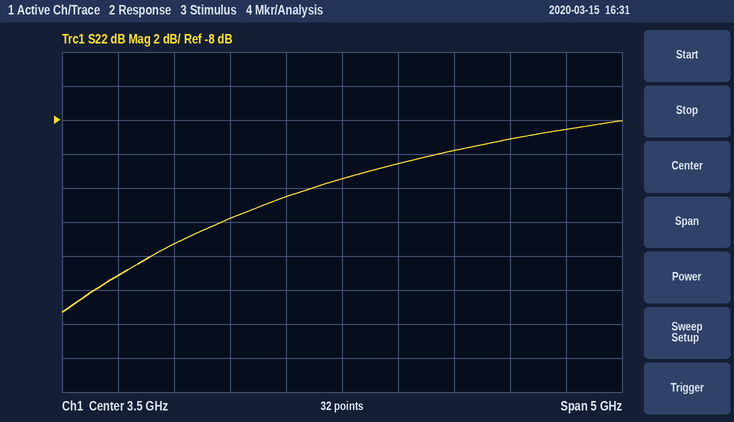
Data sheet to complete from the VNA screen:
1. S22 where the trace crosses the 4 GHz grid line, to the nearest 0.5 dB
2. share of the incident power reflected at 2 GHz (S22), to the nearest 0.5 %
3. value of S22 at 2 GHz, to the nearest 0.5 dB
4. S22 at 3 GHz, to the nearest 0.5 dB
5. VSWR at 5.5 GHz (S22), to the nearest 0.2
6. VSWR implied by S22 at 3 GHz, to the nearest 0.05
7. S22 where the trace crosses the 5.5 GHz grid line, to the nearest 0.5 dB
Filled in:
-10.5 dB
3.0 %
-15.5 dB
-12.5 dB
2.2
1.60
-8.5 dB
